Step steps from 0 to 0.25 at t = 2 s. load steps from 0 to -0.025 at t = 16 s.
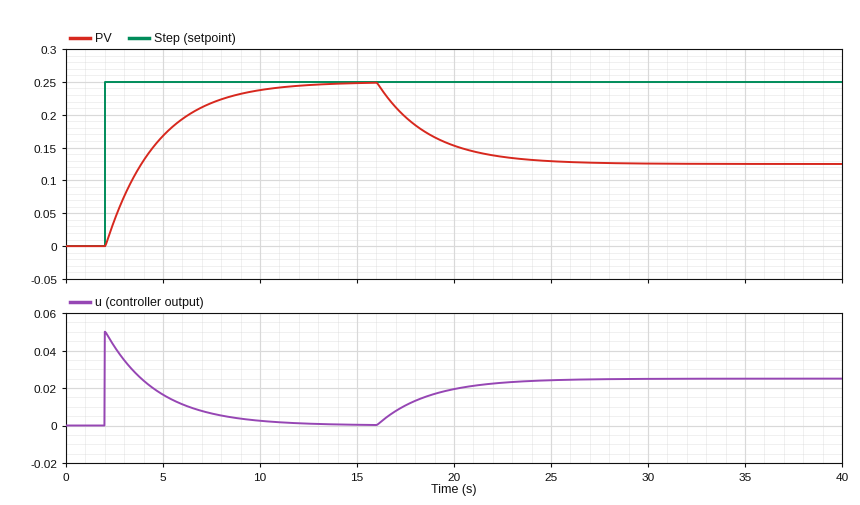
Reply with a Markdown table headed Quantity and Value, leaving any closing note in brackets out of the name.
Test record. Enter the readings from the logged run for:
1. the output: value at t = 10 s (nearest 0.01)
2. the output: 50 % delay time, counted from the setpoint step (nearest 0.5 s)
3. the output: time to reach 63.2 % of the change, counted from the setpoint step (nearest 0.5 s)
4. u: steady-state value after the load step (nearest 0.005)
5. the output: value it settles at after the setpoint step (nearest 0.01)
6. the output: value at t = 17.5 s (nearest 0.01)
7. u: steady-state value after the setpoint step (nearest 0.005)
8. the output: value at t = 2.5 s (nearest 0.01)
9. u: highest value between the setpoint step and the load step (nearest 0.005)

| Quantity | Value |
|---|---|
| the output: value at t = 10 s | 0.24 |
| the output: 50 % delay time, counted from the setpoint step | 2.0 s |
| the output: time to reach 63.2 % of the change, counted from the setpoint step | 2.5 s |
| u: steady-state value after the load step | 0.025 |
| the output: value it settles at after the setpoint step | 0.25 |
| the output: value at t = 17.5 s | 0.20 |
| u: steady-state value after the setpoint step | 0.000 |
| the output: value at t = 2.5 s | 0.04 |
| u: highest value between the setpoint step and the load step | 0.050 |
